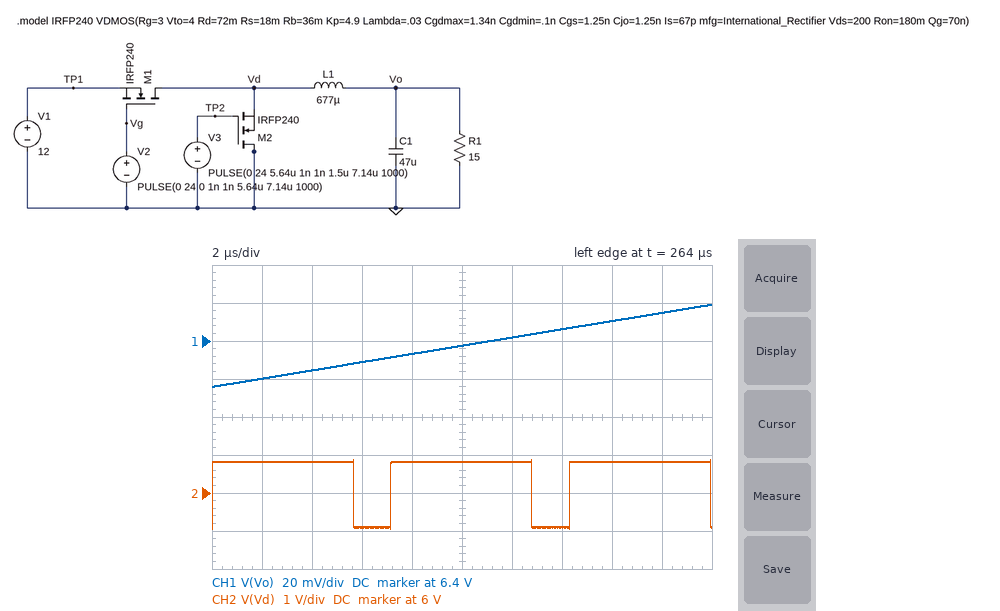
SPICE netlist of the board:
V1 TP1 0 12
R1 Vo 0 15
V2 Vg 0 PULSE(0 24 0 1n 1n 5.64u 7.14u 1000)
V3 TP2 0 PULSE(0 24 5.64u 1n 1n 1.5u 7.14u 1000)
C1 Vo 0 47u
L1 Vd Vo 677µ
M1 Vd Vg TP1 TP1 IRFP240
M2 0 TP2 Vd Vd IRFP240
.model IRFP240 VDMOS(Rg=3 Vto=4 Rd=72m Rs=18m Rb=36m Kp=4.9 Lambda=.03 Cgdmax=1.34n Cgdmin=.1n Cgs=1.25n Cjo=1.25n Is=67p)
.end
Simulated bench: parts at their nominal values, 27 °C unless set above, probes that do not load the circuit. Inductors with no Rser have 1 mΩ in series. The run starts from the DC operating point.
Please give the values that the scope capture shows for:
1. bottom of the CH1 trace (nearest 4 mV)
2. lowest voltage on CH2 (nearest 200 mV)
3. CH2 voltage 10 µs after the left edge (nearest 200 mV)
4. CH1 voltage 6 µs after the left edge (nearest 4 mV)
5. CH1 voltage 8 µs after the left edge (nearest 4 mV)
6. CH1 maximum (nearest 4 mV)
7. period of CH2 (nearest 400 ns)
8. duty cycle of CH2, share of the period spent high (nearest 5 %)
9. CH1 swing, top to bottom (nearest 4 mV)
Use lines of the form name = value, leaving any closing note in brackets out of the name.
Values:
bottom of the CH1 trace = 6.376 V
lowest voltage on CH2 = 5.0 V
CH2 voltage 10 µs after the left edge = 6.8 V
CH1 voltage 6 µs after the left edge = 6.388 V
CH1 voltage 8 µs after the left edge = 6.392 V
CH1 maximum = 6.420 V
period of CH2 = 7.2 µs
duty cycle of CH2, share of the period spent high = 80 %
CH1 swing, top to bottom = 44 mV
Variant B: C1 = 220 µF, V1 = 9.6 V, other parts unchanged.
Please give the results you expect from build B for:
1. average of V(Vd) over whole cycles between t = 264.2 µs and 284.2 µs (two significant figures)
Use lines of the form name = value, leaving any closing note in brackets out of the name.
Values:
average of V(Vd) over whole cycles between t = 264.2 µs and 284.2 µs = 5.2 V
